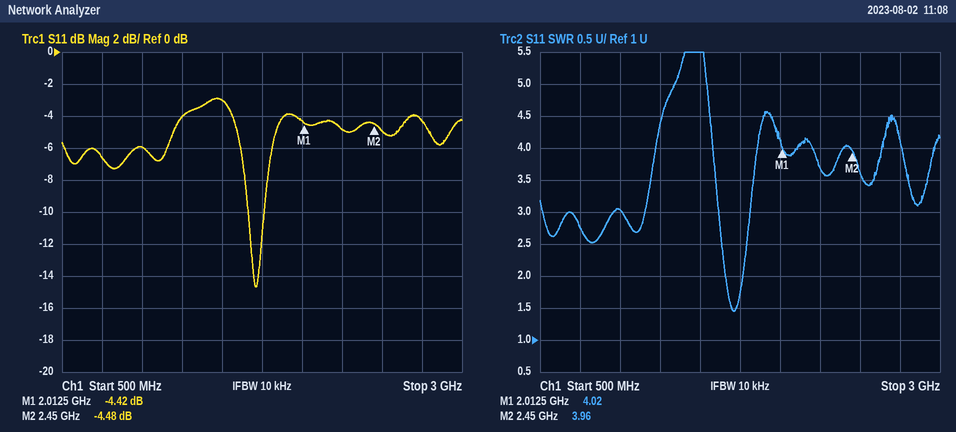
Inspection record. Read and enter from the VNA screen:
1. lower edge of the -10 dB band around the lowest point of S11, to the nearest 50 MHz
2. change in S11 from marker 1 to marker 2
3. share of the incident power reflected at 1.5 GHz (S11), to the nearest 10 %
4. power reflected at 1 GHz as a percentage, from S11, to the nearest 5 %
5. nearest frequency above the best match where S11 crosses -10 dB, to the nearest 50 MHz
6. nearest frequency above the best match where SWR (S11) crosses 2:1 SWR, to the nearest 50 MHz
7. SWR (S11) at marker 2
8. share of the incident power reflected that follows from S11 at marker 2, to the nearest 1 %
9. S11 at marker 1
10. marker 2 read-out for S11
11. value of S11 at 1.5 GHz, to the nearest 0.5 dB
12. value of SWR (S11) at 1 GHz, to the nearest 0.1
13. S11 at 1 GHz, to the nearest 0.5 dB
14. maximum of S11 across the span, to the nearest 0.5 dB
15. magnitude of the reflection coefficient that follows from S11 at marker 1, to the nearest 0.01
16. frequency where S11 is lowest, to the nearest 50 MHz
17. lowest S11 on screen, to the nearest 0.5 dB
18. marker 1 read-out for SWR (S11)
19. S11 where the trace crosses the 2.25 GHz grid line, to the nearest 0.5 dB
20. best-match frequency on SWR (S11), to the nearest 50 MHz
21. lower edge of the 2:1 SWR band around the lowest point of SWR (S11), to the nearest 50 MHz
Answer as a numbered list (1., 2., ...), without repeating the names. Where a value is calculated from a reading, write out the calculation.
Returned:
1. 1.65 GHz
2. -4.48 − (-4.42) = -0.06 dB
3. 10^(-3/10) ≈ 50 %
4. 10^(-6/10) ≈ 25 %
5. 1.75 GHz
6. 1.75 GHz
7. 3.96
8. 10^(-4.48/10) ≈ 36 %
9. -4.42 dB
10. -4.48 dB
11. -3.0 dB
12. 3.0
13. -6.0 dB
14. -3.0 dB
15. 10^(-4.42/20) ≈ 0.60
16. 1.70 GHz
17. -14.5 dB
18. 4.02
19. -5.0 dB
20. 1.70 GHz
21. 1.65 GHz
